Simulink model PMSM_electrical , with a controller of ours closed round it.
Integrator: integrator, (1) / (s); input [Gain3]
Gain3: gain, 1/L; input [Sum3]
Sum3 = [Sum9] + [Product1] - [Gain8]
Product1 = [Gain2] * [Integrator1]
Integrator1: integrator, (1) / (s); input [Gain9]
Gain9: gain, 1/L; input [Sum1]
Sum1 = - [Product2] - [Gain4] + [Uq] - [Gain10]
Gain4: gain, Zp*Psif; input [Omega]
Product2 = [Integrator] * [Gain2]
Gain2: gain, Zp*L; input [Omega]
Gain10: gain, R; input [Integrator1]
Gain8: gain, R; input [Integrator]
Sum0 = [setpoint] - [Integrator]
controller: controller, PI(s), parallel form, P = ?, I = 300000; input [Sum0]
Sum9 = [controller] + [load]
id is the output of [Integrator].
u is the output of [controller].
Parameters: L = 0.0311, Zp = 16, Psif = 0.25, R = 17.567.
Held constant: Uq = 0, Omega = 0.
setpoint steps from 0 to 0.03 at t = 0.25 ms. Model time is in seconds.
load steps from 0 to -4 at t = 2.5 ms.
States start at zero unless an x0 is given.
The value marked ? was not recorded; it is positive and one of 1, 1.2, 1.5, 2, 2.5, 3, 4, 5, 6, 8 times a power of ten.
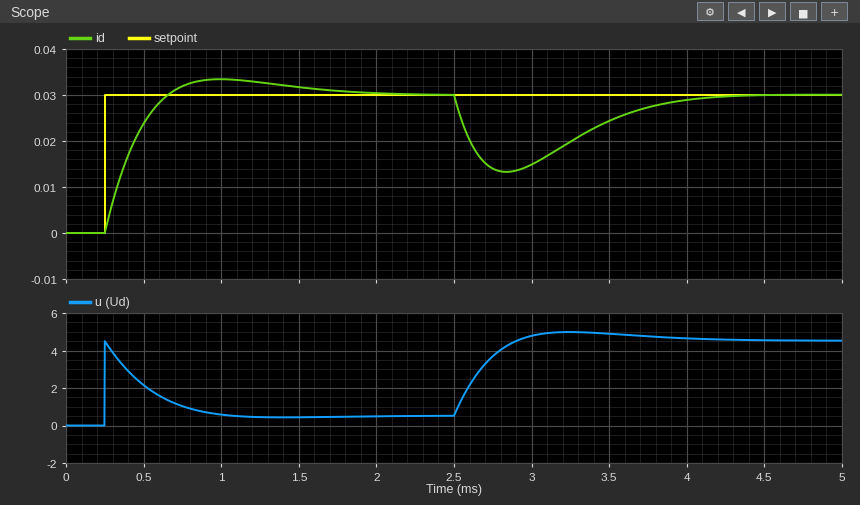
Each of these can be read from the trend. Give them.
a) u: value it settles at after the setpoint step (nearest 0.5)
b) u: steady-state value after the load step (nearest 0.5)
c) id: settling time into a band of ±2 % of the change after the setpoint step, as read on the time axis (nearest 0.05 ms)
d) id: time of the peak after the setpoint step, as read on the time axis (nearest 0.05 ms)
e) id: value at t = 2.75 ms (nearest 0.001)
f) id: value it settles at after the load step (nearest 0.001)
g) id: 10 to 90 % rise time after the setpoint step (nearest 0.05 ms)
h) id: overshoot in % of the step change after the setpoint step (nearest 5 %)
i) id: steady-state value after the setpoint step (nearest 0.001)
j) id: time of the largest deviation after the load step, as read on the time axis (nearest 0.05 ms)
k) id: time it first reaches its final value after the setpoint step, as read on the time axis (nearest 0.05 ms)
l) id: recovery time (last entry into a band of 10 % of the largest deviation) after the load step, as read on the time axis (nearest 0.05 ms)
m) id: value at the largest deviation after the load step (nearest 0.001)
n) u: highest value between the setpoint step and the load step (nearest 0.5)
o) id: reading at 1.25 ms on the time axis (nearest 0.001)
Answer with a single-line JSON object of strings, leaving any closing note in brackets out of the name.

{"u: value it settles at after the setpoint step": "0.5", "u: steady-state value after the load step": "4.5", "id: settling time into a band of ±2 % of the change after the setpoint step, as read on the time axis": "1.90 ms", "id: time of the peak after the setpoint step, as read on the time axis": "1.00 ms", "id: value at t = 2.75 ms": "0.014", "id: value it settles at after the load step": "0.030", "id: 10 to 90 % rise time after the setpoint step": "0.30 ms", "id: overshoot in % of the step change after the setpoint step": "10 %", "id: steady-state value after the setpoint step": "0.030", "id: time of the largest deviation after the load step, as read on the time axis": "2.85 ms", "id: time it first reaches its final value after the setpoint step, as read on the time axis": "0.65 ms", "id: recovery time (last entry into a band of 10 % of the largest deviation) after the load step, as read on the time axis": "3.90 ms", "id: value at the largest deviation after the load step": "0.013", "u: highest value between the setpoint step and the load step": "4.5", "id: reading at 1.25 ms on the time axis": "0.033"}
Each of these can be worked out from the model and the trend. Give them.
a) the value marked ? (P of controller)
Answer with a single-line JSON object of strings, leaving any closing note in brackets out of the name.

{"the value marked ?": "150"}
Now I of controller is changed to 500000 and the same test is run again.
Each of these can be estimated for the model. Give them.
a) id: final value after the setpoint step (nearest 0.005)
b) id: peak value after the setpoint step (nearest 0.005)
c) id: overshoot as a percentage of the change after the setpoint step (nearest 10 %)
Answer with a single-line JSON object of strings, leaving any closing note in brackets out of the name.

{"id: final value after the setpoint step": "0.030", "id: peak value after the setpoint step": "0.035", "id: overshoot as a percentage of the change after the setpoint step": "20 %"}
